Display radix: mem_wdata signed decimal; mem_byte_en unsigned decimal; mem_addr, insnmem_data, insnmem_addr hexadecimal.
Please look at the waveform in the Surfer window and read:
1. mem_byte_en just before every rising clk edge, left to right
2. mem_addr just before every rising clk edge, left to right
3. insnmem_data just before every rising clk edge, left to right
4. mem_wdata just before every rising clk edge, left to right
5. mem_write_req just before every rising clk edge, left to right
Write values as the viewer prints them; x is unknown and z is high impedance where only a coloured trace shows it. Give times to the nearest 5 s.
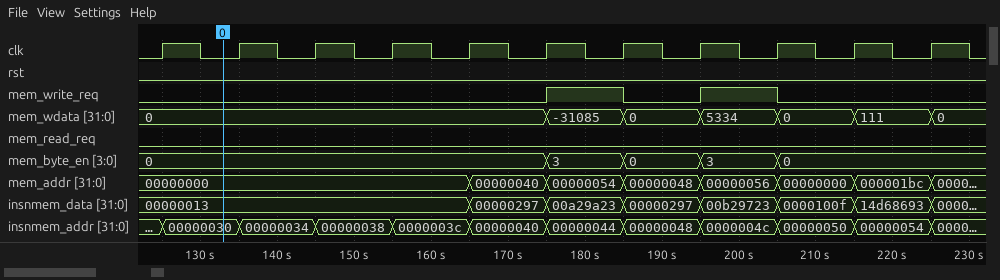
0, 0, 0, 0, 0, 0, 3, 0, 3, 0, 0
00000000, 00000000, 00000000, 00000000, 00000000, 00000040, 00000054, 00000048, 00000056, 00000000, 000001bc
00000013, 00000013, 00000013, 00000013, 00000013, 00000297, 00a29a23, 00000297, 00b29723, 0000100f, 14d68693
0, 0, 0, 0, 0, 0, -31085, 0, 5334, 0, 111
0 0 0 0 0 0 1 0 1 0 0
